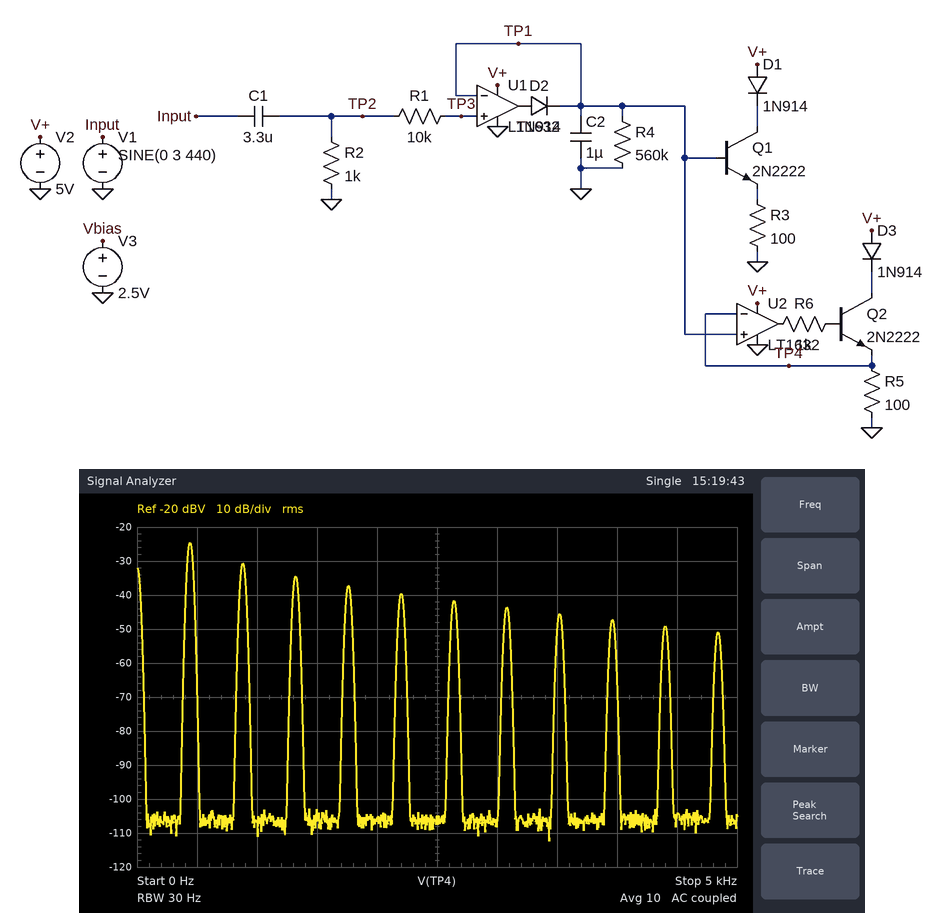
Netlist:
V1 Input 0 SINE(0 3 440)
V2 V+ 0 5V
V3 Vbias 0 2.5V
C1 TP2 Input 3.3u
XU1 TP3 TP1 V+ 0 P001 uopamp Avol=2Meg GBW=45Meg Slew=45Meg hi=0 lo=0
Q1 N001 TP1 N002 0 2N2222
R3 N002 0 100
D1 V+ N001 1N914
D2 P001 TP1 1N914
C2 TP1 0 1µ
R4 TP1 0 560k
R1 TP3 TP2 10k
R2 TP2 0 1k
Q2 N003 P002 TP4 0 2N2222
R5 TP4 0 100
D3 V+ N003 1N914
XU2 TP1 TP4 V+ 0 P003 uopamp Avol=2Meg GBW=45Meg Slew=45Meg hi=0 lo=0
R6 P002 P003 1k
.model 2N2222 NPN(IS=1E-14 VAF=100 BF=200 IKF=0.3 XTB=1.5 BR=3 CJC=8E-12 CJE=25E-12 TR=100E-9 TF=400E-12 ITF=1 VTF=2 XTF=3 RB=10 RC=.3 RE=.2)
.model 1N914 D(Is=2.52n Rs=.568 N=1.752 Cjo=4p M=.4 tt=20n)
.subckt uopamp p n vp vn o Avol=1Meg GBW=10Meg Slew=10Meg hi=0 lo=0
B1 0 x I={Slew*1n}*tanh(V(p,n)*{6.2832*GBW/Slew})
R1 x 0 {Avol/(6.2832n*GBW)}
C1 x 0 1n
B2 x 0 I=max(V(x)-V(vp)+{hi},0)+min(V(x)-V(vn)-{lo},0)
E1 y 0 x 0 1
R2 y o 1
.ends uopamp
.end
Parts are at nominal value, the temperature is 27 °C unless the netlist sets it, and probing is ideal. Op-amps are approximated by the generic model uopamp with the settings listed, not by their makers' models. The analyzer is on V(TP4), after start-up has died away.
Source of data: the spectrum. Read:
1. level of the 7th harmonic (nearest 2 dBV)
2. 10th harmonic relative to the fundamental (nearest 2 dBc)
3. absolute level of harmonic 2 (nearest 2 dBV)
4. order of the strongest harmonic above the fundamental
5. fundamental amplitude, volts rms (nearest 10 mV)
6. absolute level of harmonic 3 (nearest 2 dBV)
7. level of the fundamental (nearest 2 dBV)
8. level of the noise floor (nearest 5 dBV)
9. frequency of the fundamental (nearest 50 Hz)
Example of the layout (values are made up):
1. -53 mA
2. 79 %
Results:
1. -44 dBV
2. -24 dBc
3. -30 dBV
4. 2
5. 60 mV
6. -34 dBV
7. -24 dBV
8. -105 dBV
9. 450 Hz
